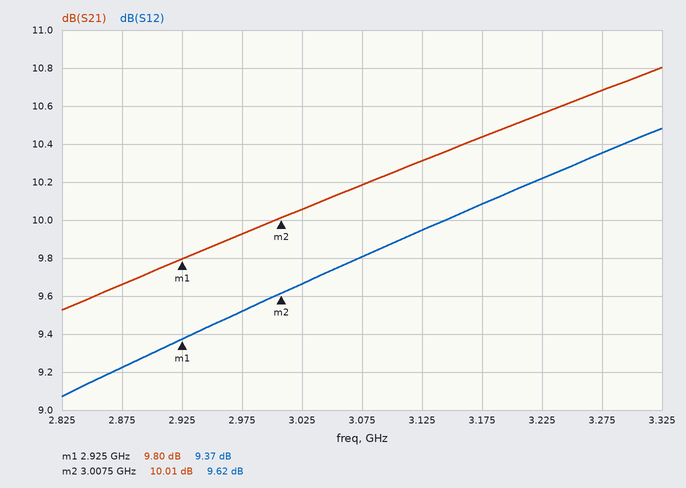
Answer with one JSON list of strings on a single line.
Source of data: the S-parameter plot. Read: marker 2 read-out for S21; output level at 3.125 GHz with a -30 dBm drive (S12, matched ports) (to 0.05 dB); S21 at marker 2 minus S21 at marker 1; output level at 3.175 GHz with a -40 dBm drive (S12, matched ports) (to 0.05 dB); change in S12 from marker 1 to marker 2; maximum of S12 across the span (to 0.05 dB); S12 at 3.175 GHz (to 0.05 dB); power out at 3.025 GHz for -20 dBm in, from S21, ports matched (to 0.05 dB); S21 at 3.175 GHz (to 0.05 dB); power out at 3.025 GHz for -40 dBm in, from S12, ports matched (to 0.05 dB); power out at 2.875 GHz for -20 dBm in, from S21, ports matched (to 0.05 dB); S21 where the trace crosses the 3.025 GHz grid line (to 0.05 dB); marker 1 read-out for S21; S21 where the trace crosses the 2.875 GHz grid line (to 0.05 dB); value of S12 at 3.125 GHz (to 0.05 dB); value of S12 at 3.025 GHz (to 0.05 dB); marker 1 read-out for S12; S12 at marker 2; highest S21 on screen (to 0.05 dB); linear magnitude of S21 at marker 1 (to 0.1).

["10.01 dB", "-20.05 dBm", "0.21 dB", "-29.90 dBm", "0.25 dB", "10.50 dB", "10.10 dB", "-9.95 dBm", "10.45 dB", "-30.35 dBm", "-10.35 dBm", "10.05 dB", "9.80 dB", "9.65 dB", "9.95 dB", "9.65 dB", "9.37 dB", "9.62 dB", "10.80 dB", "3.1"]
